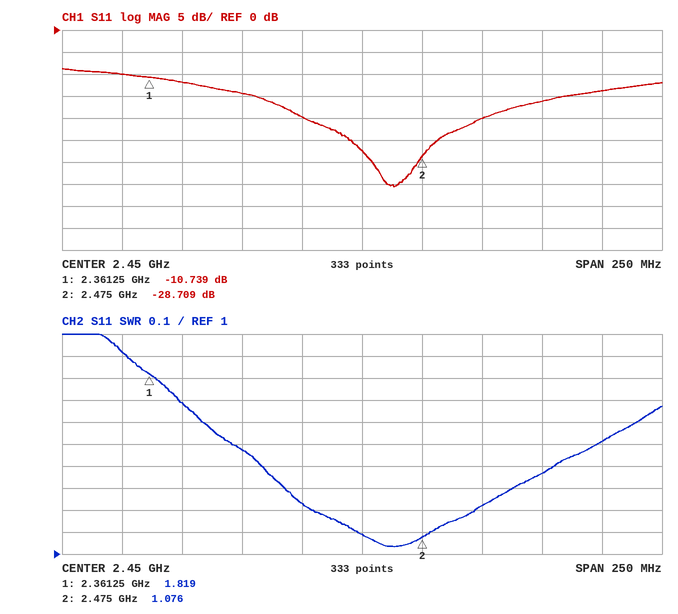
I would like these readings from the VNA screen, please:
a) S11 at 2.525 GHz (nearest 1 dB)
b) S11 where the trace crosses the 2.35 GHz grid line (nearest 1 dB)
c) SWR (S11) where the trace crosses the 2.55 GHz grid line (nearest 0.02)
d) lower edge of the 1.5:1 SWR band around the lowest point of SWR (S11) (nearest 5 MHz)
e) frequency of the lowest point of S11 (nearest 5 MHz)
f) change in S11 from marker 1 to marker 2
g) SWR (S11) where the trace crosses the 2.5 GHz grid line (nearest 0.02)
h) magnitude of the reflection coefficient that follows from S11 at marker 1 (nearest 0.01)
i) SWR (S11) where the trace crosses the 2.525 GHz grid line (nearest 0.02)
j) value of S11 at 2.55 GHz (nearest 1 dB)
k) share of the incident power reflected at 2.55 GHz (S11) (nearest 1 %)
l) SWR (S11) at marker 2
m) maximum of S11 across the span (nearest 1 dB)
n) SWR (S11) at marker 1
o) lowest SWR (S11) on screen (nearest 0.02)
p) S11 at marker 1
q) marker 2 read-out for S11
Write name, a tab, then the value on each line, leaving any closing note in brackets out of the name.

S11 at 2.525 GHz	-16 dB
S11 where the trace crosses the 2.35 GHz grid line	-10 dB
SWR (S11) where the trace crosses the 2.55 GHz grid line	1.52
lower edge of the 1.5:1 SWR band around the lowest point of SWR (S11)	2.395 GHz
frequency of the lowest point of S11	2.465 GHz
change in S11 from marker 1 to marker 2	-17.970 dB
SWR (S11) where the trace crosses the 2.5 GHz grid line	1.22
magnitude of the reflection coefficient that follows from S11 at marker 1	0.29
SWR (S11) where the trace crosses the 2.525 GHz grid line	1.36
value of S11 at 2.55 GHz	-14 dB
share of the incident power reflected at 2.55 GHz (S11)	4 %
SWR (S11) at marker 2	1.076
maximum of S11 across the span	-9 dB
SWR (S11) at marker 1	1.819
lowest SWR (S11) on screen	1.04
S11 at marker 1	-10.739 dB
marker 2 read-out for S11	-28.709 dB
